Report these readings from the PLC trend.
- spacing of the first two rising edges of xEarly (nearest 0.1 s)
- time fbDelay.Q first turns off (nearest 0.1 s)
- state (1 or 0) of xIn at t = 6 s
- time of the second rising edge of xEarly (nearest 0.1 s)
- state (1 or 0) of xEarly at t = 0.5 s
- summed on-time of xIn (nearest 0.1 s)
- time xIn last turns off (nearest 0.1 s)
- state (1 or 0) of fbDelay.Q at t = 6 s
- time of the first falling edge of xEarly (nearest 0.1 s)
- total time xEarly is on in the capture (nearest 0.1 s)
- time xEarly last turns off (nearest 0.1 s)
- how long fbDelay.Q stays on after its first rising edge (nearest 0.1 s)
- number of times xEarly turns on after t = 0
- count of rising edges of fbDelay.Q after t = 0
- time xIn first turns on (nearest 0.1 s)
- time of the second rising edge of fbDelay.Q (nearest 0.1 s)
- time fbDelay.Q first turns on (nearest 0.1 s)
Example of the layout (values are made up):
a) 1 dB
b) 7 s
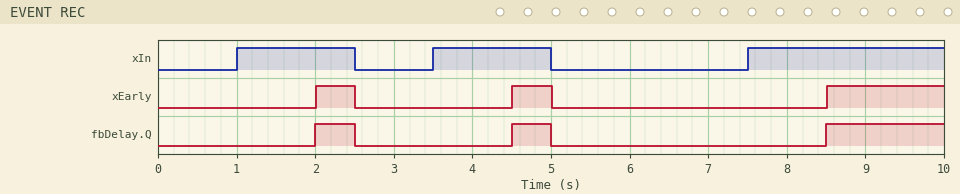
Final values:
a) 2.5 s
b) 2.5 s
c) 0
d) 4.5 s
e) 0
f) 5.5 s
g) 5.0 s
h) 0
i) 2.5 s
j) 2.5 s
k) 5.0 s
l) 0.5 s
m) 3
n) 3
o) 1.0 s
p) 4.5 s
q) 2.0 s
